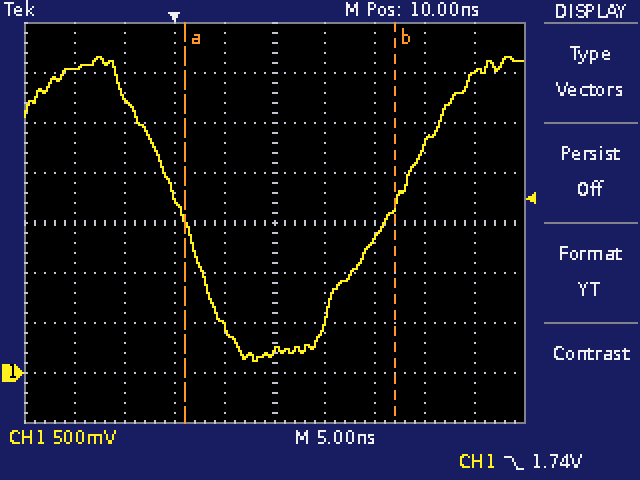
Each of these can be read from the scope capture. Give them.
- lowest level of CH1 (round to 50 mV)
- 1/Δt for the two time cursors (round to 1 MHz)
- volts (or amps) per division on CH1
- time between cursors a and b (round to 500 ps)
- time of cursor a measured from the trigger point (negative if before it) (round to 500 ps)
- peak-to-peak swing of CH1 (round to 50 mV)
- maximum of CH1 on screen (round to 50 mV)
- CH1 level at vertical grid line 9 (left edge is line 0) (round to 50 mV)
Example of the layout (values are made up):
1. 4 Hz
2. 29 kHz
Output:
1. 100 mV
2. 48 MHz
3. 500 mV
4. 21.0 ns
5. +1.0 ns
6. 3.05 V
7. 3.15 V
8. 3.00 V
